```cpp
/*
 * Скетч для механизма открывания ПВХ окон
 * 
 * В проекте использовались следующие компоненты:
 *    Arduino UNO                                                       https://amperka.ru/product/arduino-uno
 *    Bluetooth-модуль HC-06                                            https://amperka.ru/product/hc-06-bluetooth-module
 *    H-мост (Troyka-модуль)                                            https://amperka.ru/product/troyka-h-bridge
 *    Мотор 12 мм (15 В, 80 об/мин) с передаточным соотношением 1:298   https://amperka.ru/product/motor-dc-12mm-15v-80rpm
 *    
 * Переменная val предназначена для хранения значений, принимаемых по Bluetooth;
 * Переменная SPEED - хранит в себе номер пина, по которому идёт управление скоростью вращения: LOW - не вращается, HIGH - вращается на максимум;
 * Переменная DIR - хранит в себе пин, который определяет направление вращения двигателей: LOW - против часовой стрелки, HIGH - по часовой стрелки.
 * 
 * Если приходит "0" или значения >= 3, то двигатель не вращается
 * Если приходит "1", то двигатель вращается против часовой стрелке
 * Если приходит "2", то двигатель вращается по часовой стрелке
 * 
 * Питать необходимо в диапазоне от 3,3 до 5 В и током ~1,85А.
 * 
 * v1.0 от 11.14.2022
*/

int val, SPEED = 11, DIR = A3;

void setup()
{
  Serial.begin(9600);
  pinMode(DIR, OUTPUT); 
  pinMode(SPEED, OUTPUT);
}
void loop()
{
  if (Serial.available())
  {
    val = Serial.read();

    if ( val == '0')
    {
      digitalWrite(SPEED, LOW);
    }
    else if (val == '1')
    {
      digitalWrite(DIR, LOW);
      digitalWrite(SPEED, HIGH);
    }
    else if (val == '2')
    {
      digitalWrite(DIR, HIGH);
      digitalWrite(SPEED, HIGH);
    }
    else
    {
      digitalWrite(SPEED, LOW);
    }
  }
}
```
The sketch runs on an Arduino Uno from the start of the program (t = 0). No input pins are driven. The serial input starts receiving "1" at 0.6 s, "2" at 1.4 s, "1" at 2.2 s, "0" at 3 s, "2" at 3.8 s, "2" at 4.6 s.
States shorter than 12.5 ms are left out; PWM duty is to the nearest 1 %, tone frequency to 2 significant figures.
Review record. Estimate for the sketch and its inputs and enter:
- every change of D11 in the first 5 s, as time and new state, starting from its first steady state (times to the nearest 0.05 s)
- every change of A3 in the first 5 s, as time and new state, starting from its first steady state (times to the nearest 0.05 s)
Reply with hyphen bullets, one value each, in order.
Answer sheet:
- 0 s low; 0.6 s high; 3 s low; 3.8 s high
- 0 s low; 1.4 s high; 2.2 s low; 3.8 s high
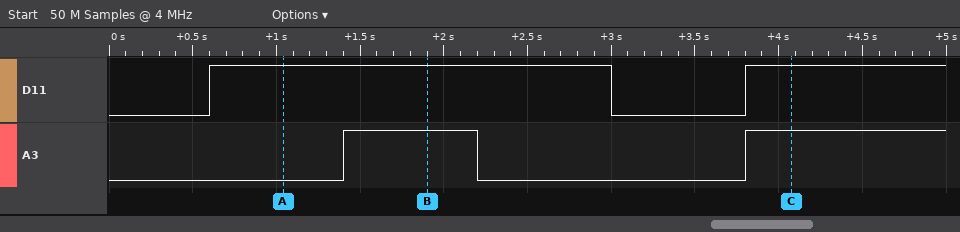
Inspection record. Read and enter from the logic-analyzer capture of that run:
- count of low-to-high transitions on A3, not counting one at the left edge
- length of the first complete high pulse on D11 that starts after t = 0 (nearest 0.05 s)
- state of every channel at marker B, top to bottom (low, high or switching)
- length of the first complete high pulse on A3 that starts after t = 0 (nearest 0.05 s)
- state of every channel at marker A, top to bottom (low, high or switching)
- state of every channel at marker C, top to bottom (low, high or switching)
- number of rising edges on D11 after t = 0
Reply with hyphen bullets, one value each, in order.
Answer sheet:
- 2
- 2.40 s
- D11 high, A3 high
- 0.80 s
- D11 high, A3 low
- D11 high, A3 high
- 2
